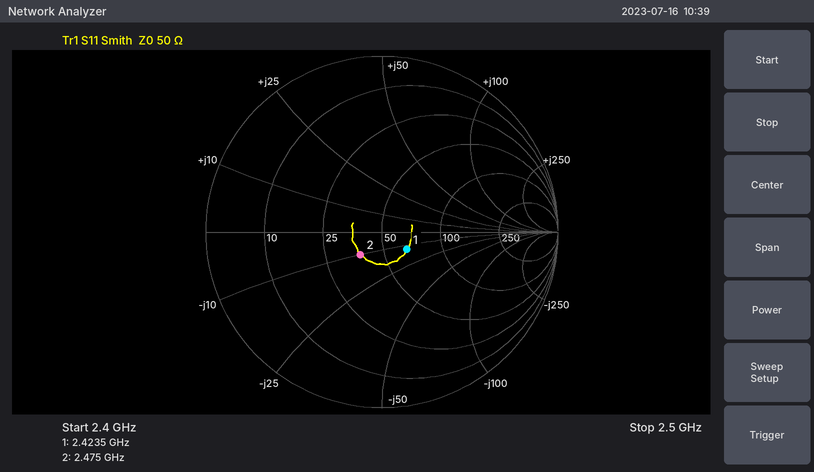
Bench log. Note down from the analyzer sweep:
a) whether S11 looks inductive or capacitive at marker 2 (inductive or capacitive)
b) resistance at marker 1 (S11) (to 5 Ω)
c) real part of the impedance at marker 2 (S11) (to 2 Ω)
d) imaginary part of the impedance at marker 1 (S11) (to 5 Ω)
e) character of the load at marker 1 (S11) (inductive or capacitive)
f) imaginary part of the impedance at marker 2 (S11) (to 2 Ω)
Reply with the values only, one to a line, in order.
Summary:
capacitive
65 Ω
38 Ω
-15 Ω
capacitive
-10 Ω
